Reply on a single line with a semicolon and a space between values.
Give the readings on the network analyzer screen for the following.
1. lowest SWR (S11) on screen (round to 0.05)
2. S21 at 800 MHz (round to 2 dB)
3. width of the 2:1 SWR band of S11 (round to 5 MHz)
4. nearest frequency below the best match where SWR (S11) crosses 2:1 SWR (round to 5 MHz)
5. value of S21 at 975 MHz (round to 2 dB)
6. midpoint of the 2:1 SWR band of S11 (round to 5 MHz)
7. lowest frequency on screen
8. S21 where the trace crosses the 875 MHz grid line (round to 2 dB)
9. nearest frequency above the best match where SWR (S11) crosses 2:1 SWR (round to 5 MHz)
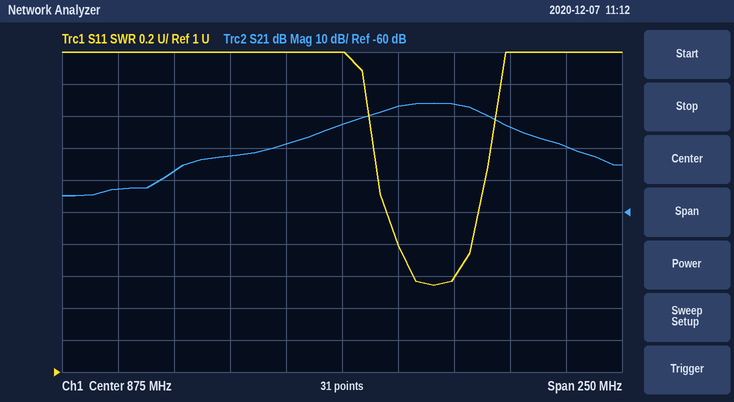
1.55; -48 dB; 40 MHz; 895 MHz; -40 dB; 915 MHz; 750 MHz; -32 dB; 935 MHz
